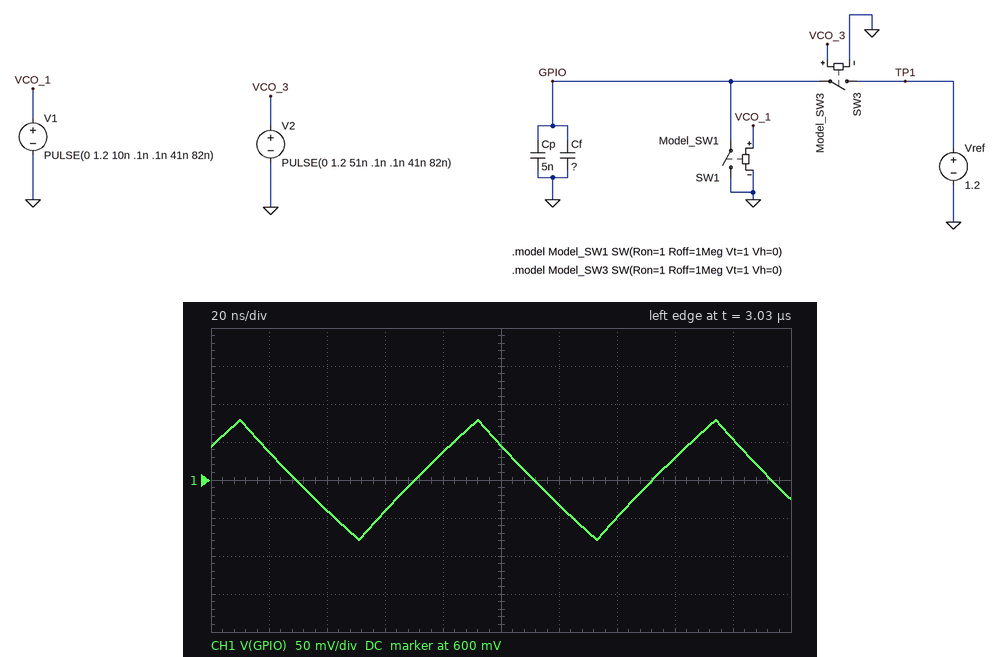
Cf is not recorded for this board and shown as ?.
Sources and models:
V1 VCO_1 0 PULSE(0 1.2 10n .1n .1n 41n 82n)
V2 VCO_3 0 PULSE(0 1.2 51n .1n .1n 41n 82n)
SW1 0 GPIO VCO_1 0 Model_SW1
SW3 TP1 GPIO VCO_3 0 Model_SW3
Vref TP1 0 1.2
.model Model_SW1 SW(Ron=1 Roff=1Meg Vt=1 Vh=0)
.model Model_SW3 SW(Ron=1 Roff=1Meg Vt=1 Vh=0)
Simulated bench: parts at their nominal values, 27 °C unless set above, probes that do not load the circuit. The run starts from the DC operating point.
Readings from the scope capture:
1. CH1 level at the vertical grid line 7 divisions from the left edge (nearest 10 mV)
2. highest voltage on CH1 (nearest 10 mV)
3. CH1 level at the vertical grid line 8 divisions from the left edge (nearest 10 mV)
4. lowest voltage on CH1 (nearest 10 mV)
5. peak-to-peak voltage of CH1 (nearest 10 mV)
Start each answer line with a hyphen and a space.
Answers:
- 550 mV
- 680 mV
- 630 mV
- 520 mV
- 160 mV
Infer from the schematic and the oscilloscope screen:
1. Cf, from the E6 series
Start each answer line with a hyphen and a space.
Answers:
- 150 nF
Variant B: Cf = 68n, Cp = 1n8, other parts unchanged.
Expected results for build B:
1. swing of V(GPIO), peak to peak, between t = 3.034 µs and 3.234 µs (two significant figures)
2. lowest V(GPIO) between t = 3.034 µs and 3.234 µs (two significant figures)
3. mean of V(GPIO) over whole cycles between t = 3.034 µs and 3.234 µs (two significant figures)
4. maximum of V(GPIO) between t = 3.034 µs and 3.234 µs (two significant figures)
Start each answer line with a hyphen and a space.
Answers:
- 340 mV
- 430 mV
- 600 mV
- 770 mV
